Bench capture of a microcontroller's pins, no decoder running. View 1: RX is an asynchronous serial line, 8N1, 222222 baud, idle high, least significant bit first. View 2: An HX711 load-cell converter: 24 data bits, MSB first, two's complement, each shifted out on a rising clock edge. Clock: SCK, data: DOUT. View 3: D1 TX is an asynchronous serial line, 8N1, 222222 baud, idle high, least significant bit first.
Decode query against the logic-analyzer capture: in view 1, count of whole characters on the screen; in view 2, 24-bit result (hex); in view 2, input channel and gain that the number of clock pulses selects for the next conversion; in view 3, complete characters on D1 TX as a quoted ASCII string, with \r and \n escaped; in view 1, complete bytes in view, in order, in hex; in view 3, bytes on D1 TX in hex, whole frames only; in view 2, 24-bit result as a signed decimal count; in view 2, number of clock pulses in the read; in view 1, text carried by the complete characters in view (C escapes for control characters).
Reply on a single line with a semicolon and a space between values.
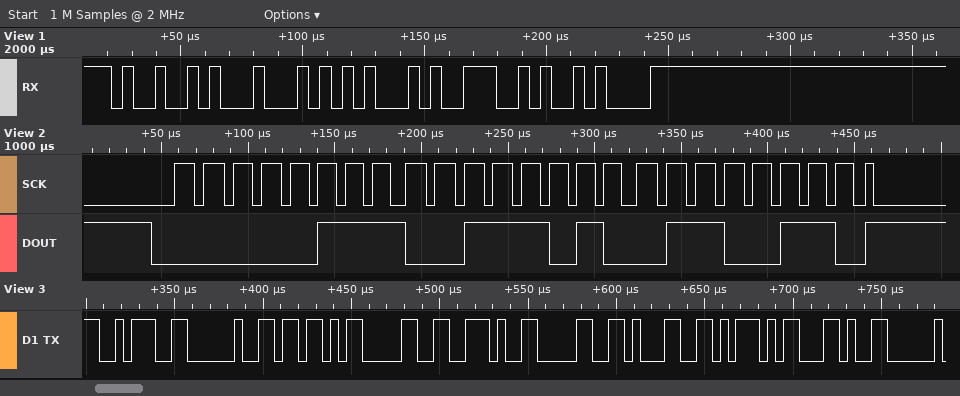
5; 0x073A66; channel A, gain 128; ": [0.01],"; 0x49 0x44 0x45 0x4E 0x0A; 3A 20 5B 30 2E 30 31 5D 2C; 473702; 25; "IDEN\n"
